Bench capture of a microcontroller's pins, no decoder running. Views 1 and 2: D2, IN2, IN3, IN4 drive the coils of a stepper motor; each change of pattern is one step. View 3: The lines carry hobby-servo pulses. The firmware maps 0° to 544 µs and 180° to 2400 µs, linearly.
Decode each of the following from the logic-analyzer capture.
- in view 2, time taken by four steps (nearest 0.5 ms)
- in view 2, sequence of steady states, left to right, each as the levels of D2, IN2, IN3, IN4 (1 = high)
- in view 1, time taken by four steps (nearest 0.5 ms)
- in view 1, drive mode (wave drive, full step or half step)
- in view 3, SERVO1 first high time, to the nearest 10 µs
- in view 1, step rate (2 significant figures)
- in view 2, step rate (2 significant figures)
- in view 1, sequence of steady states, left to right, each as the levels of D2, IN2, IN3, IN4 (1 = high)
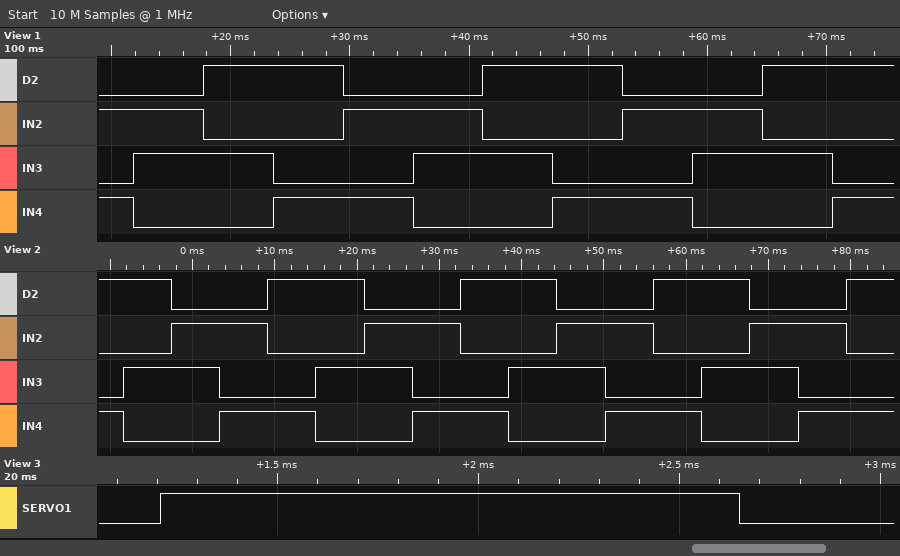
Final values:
23.5 ms
1001 1010 0110 0101 1001 1010 0110 0101 1001 1010 0110 0101 1001 1010 0110 0101 1001
23.5 ms
full step
1440 µs
170 steps/s
170 steps/s
0101 0110 1010 1001 0101 0110 1010 1001 0101 0110 1010 1001
